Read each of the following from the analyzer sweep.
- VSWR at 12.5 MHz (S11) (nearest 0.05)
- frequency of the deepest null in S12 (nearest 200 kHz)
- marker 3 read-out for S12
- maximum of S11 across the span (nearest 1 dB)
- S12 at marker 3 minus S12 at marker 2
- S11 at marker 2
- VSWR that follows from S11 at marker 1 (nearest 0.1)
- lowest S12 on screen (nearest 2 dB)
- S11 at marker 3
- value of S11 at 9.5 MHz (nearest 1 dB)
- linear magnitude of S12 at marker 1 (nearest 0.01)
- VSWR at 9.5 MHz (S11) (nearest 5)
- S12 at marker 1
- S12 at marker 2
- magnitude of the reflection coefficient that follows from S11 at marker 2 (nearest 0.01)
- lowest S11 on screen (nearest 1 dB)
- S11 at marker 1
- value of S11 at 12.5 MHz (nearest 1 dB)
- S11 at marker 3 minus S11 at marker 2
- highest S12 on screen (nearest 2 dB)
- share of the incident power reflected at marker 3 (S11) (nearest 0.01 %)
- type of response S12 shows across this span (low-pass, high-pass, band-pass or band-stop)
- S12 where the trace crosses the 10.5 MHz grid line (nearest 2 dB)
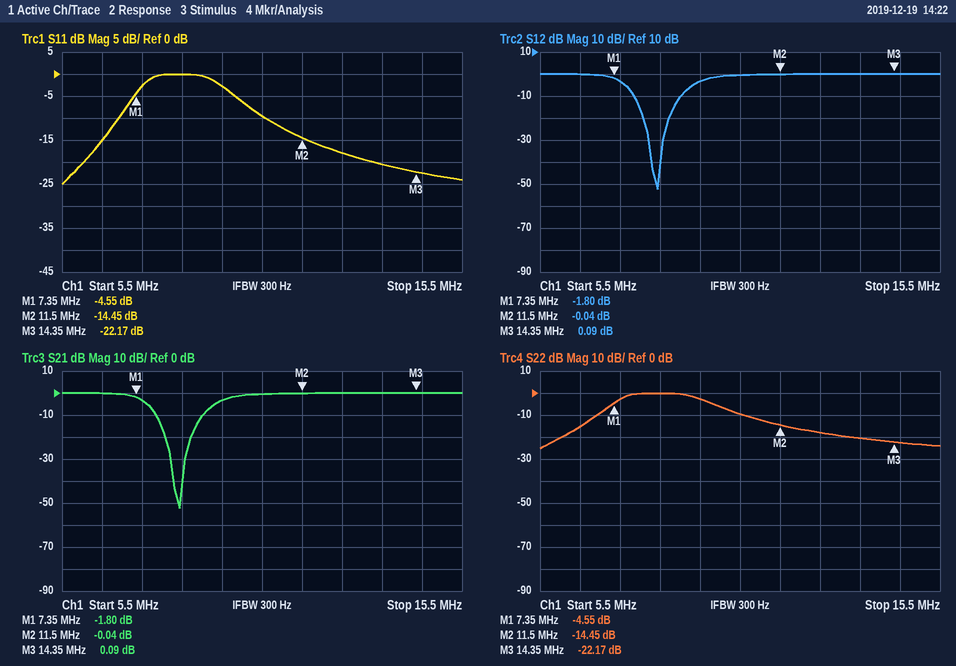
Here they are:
1.30
8.4 MHz
0.09 dB
0 dB
0.13 dB
-14.45 dB
3.9
-52 dB
-22.17 dB
-3 dB
0.81
5
-1.80 dB
-0.04 dB
0.19
-25 dB
-4.55 dB
-18 dB
-7.72 dB
0 dB
0.61 %
band-stop
0 dB
